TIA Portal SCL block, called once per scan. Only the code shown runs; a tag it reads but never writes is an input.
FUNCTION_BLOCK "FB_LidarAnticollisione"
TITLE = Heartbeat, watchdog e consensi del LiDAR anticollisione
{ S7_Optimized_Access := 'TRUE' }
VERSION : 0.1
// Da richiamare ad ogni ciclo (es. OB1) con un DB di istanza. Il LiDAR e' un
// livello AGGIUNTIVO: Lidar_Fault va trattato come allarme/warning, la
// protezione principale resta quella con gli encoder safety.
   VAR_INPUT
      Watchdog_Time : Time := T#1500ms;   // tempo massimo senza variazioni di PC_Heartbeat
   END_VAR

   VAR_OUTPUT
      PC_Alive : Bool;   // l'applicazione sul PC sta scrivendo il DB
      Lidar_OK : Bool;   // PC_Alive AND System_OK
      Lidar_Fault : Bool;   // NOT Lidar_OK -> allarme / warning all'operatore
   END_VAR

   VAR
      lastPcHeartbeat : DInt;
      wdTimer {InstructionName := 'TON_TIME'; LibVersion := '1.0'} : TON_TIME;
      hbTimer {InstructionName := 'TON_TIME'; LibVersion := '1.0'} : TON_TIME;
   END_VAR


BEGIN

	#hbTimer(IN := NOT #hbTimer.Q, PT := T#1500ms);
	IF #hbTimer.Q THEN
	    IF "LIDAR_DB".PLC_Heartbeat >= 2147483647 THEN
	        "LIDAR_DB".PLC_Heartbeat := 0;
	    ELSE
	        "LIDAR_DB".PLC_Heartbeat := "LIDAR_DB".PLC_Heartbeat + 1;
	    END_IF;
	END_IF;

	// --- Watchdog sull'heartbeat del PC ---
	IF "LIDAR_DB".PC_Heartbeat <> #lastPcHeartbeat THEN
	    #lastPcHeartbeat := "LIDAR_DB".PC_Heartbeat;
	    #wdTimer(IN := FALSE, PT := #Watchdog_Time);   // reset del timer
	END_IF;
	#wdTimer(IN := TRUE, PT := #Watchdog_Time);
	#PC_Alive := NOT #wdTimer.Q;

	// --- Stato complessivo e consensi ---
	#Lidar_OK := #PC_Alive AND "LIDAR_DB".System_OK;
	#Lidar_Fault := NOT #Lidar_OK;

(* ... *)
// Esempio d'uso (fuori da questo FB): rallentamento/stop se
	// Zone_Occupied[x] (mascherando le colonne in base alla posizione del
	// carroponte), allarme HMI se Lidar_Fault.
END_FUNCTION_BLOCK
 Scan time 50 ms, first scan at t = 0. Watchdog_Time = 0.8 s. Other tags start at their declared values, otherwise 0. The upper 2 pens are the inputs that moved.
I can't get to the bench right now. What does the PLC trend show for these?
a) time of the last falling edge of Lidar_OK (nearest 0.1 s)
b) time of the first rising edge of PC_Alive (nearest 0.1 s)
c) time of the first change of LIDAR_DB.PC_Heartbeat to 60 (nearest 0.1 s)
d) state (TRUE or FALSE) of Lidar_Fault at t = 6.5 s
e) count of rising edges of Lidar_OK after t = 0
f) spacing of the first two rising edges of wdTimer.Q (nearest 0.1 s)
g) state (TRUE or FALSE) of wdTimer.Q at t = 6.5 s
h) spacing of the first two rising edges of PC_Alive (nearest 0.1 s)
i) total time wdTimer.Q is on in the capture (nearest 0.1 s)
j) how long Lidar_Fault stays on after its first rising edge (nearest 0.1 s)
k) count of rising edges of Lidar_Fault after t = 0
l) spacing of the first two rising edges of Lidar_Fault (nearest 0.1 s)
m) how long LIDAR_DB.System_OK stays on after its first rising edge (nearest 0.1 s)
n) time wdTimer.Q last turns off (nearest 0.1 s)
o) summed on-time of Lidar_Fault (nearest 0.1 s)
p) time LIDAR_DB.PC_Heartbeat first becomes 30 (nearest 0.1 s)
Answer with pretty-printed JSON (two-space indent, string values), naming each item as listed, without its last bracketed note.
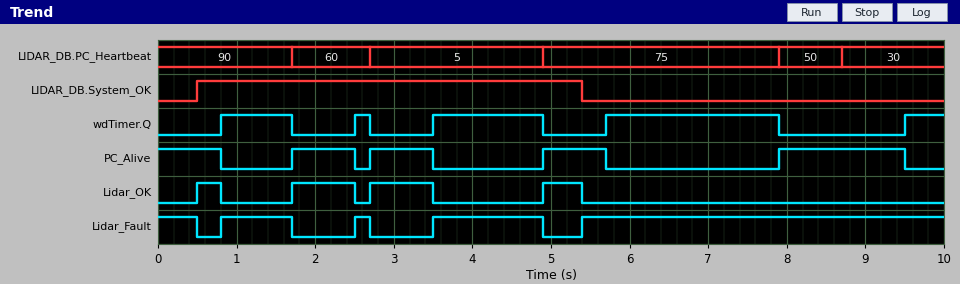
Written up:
{
  "time of the last falling edge of Lidar_OK": "5.4 s",
  "time of the first rising edge of PC_Alive": "1.7 s",
  "time of the first change of LIDAR_DB.PC_Heartbeat to 60": "1.7 s",
  "state (TRUE or FALSE) of Lidar_Fault at t = 6.5 s": "TRUE",
  "count of rising edges of Lidar_OK after t = 0": "4",
  "spacing of the first two rising edges of wdTimer.Q": "1.7 s",
  "state (TRUE or FALSE) of wdTimer.Q at t = 6.5 s": "TRUE",
  "spacing of the first two rising edges of PC_Alive": "1.0 s",
  "total time wdTimer.Q is on in the capture": "5.2 s",
  "how long Lidar_Fault stays on after its first rising edge": "0.9 s",
  "count of rising edges of Lidar_Fault after t = 0": "4",
  "spacing of the first two rising edges of Lidar_Fault": "1.7 s",
  "how long LIDAR_DB.System_OK stays on after its first rising edge": "4.9 s",
  "time wdTimer.Q last turns off": "7.9 s",
  "summed on-time of Lidar_Fault": "7.6 s",
  "time LIDAR_DB.PC_Heartbeat first becomes 30": "8.7 s"
}
